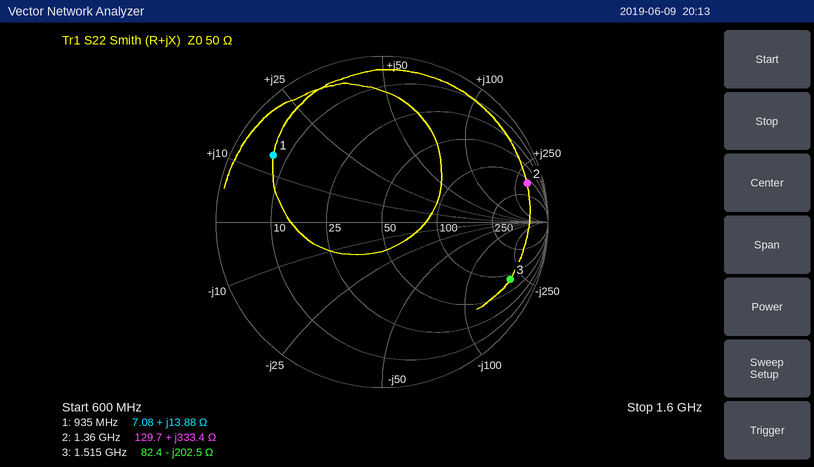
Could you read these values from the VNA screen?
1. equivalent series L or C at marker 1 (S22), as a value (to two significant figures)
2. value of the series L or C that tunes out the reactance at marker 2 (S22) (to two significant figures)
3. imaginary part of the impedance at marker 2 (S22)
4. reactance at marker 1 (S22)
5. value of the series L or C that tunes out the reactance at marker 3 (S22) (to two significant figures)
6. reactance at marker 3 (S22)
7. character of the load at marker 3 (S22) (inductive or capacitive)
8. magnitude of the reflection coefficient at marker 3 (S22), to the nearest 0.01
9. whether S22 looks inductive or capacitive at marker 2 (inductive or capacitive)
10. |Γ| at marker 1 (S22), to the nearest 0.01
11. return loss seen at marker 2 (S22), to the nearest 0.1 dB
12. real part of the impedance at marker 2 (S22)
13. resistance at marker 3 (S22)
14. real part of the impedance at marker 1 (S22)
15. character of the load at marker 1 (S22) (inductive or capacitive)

2.4 nH
350 fF
+333.4 Ω
+13.88 Ω
21 nH
-202.5 Ω
capacitive
0.85
inductive
0.77
0.9 dB
129.7 Ω
82.4 Ω
7.08 Ω
inductive
